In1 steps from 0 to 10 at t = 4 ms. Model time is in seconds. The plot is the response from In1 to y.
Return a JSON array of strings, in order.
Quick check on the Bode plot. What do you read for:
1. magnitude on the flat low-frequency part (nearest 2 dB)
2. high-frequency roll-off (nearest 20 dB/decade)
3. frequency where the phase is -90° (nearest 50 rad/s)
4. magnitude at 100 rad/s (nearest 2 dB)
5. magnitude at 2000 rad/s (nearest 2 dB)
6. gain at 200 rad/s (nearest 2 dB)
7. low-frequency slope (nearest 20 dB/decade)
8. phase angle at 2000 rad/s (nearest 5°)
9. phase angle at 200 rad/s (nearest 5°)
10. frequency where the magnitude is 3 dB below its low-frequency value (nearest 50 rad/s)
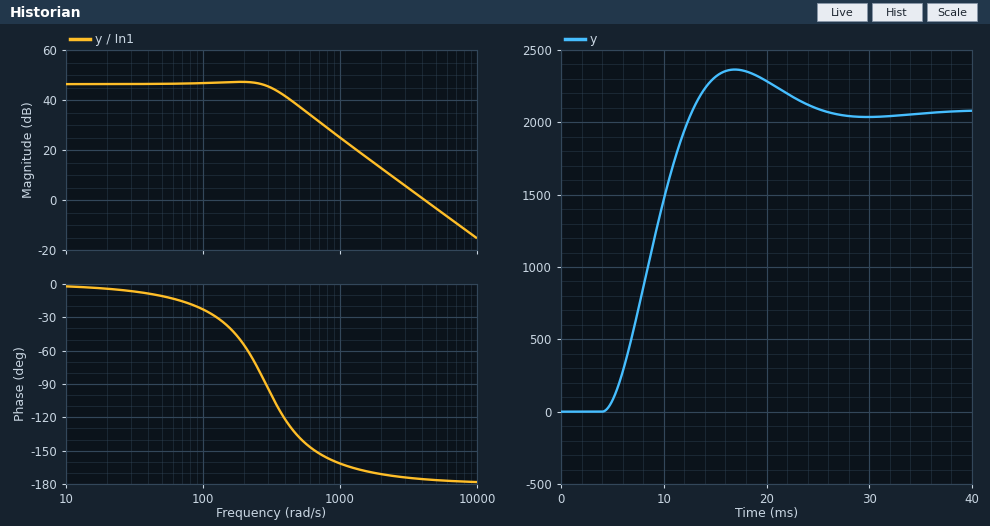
["46 dB", "-40 dB/decade", "300 rad/s", "46 dB", "12 dB", "48 dB", "0 dB/decade", "-170°", "-55°", "350 rad/s"]
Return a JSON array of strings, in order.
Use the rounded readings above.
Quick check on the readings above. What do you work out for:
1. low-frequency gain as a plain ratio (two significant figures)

["200"]
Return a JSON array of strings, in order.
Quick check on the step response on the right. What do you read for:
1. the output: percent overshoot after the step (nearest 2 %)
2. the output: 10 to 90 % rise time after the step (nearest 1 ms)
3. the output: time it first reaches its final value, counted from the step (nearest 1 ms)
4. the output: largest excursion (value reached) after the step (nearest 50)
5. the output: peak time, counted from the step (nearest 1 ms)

["14 %", "6 ms", "9 ms", "2350", "13 ms"]
